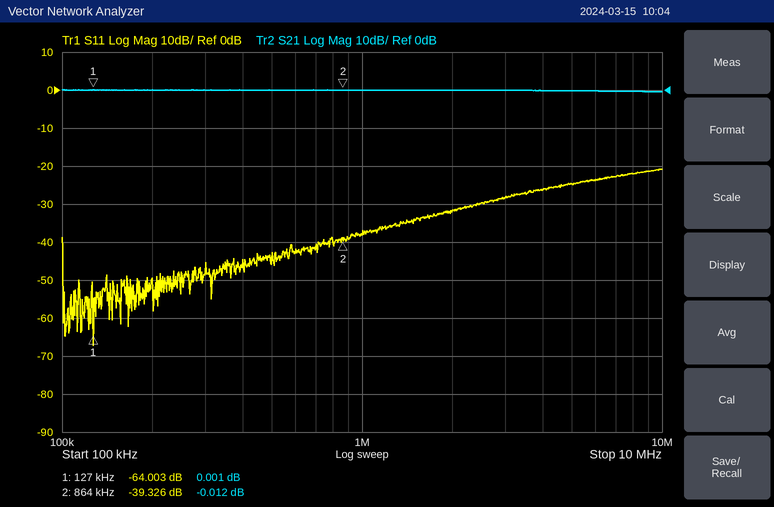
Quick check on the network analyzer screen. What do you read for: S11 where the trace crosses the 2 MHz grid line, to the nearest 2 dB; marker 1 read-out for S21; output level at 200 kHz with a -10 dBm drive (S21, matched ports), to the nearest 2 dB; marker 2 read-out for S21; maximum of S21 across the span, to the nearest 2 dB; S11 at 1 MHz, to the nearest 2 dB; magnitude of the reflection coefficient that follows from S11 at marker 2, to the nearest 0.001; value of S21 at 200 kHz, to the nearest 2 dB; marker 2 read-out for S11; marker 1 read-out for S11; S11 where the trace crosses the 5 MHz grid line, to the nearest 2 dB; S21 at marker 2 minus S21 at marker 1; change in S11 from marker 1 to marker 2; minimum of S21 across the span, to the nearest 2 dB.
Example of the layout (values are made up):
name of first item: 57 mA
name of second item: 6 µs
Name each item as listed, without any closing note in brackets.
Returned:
S11 where the trace crosses the 2 MHz grid line, to the nearest 2 dB: -32 dB
marker 1 read-out for S21: 0.001 dB
output level at 200 kHz with a -10 dBm drive (S21, matched ports), to the nearest 2 dB: -10 dBm
marker 2 read-out for S21: -0.012 dB
maximum of S21 across the span, to the nearest 2 dB: 0 dB
S11 at 1 MHz, to the nearest 2 dB: -38 dB
magnitude of the reflection coefficient that follows from S11 at marker 2, to the nearest 0.001: 0.011
value of S21 at 200 kHz, to the nearest 2 dB: 0 dB
marker 2 read-out for S11: -39.326 dB
marker 1 read-out for S11: -64.003 dB
S11 where the trace crosses the 5 MHz grid line, to the nearest 2 dB: -24 dB
S21 at marker 2 minus S21 at marker 1: -0.013 dB
change in S11 from marker 1 to marker 2: 24.677 dB
minimum of S21 across the span, to the nearest 2 dB: 0 dB
